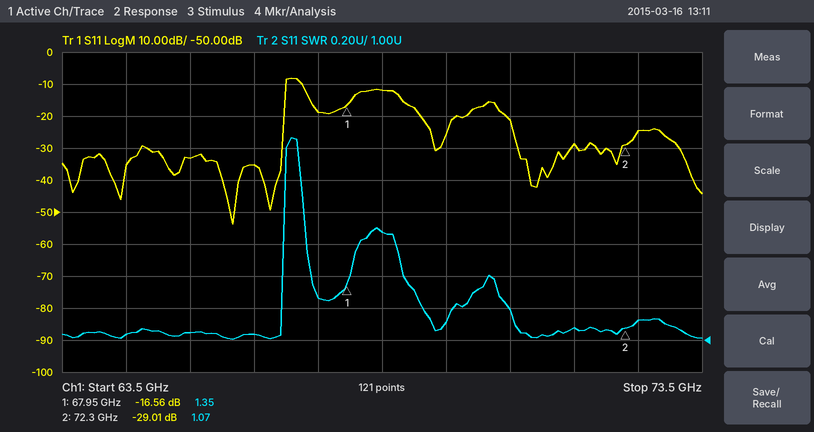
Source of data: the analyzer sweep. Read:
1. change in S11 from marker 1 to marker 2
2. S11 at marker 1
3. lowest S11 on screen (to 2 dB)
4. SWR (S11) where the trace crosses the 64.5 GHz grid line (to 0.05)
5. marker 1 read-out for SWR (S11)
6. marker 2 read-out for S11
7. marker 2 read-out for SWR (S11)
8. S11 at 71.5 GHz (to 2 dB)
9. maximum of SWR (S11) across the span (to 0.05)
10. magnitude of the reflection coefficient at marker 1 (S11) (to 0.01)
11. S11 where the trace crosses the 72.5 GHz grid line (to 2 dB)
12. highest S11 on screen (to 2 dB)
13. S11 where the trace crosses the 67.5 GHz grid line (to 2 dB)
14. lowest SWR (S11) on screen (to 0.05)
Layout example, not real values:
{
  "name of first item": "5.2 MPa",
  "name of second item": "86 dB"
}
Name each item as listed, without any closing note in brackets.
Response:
{
  "change in S11 from marker 1 to marker 2": "-12.45 dB",
  "S11 at marker 1": "-16.56 dB",
  "lowest S11 on screen": "-54 dB",
  "SWR (S11) where the trace crosses the 64.5 GHz grid line": "1.05",
  "marker 1 read-out for SWR": "1.35",
  "marker 2 read-out for S11": "-29.01 dB",
  "marker 2 read-out for SWR": "1.07",
  "S11 at 71.5 GHz": "-28 dB",
  "maximum of SWR (S11) across the span": "2.25",
  "magnitude of the reflection coefficient at marker 1 (S11)": "0.15",
  "S11 where the trace crosses the 72.5 GHz grid line": "-24 dB",
  "highest S11 on screen": "-8 dB",
  "S11 where the trace crosses the 67.5 GHz grid line": "-18 dB",
  "lowest SWR (S11) on screen": "1.00"
}
